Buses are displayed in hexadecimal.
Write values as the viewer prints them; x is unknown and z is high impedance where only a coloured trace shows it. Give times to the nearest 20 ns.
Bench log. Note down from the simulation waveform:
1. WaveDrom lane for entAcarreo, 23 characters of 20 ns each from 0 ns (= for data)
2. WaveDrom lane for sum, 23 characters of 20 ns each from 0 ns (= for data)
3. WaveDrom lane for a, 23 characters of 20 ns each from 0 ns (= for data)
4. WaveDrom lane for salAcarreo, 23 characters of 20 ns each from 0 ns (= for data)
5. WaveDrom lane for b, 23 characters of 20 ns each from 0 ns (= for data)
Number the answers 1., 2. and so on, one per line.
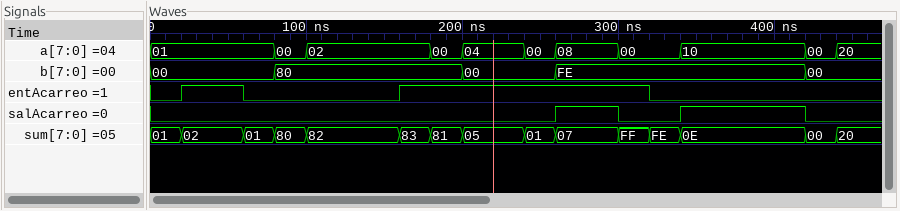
1. {name: 'entAcarreo', wave: '01.0....1.......0......'}
2. {name: 'sum', wave: '==.===..===.==.===...==', data: '01 02 01 80 82 83 81 05 01 07 FF FE 0E 00 20'}
3. {name: 'a', wave: '=...==...==.==.=.=...==', data: '01 00 02 00 04 00 08 00 10 00 20'}
4. {name: 'salAcarreo', wave: '0............1.0.1...0.'}
5. {name: 'b', wave: '=...=.....=..=.......=.', data: '00 80 00 FE 00'}
